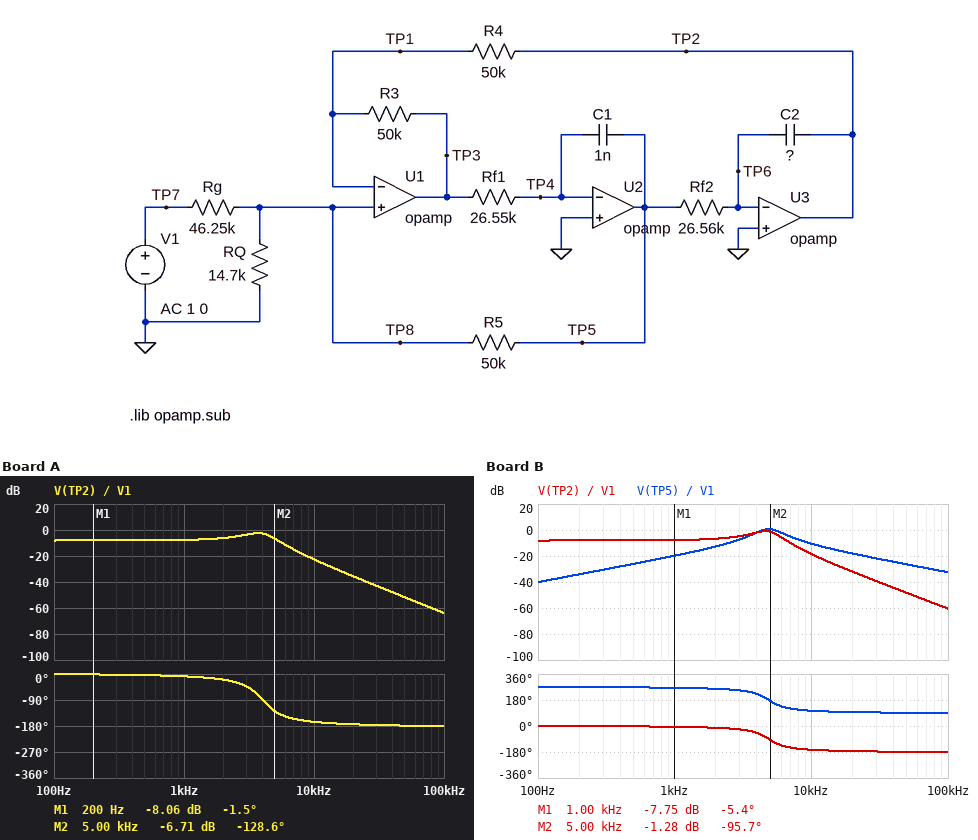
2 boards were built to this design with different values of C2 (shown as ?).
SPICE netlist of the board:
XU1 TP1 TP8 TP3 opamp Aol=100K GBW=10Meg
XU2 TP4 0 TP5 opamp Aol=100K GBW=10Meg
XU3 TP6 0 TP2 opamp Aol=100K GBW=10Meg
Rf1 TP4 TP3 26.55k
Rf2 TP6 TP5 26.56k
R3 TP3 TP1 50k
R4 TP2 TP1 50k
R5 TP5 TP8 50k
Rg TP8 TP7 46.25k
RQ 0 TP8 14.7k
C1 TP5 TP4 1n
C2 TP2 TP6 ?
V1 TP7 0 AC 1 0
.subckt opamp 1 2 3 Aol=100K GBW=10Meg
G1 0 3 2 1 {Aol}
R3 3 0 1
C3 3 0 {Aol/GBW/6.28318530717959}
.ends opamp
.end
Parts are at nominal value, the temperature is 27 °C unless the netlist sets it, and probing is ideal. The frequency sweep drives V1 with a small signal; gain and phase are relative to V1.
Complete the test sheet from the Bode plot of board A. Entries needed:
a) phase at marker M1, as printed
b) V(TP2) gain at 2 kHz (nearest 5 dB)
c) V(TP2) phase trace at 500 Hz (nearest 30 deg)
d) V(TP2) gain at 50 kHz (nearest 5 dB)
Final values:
-1.5 deg
-5 dB
0 deg
-50 dB
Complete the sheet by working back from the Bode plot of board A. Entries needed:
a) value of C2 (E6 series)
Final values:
2.2 nF
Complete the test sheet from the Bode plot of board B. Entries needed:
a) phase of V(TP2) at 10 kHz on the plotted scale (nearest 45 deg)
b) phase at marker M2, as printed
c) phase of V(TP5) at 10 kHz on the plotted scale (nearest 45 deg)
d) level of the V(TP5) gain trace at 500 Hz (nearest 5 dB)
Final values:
-180 deg
-95.7 deg
90 deg
-25 dB
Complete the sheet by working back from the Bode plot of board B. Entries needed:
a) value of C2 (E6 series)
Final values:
1.5 nF
